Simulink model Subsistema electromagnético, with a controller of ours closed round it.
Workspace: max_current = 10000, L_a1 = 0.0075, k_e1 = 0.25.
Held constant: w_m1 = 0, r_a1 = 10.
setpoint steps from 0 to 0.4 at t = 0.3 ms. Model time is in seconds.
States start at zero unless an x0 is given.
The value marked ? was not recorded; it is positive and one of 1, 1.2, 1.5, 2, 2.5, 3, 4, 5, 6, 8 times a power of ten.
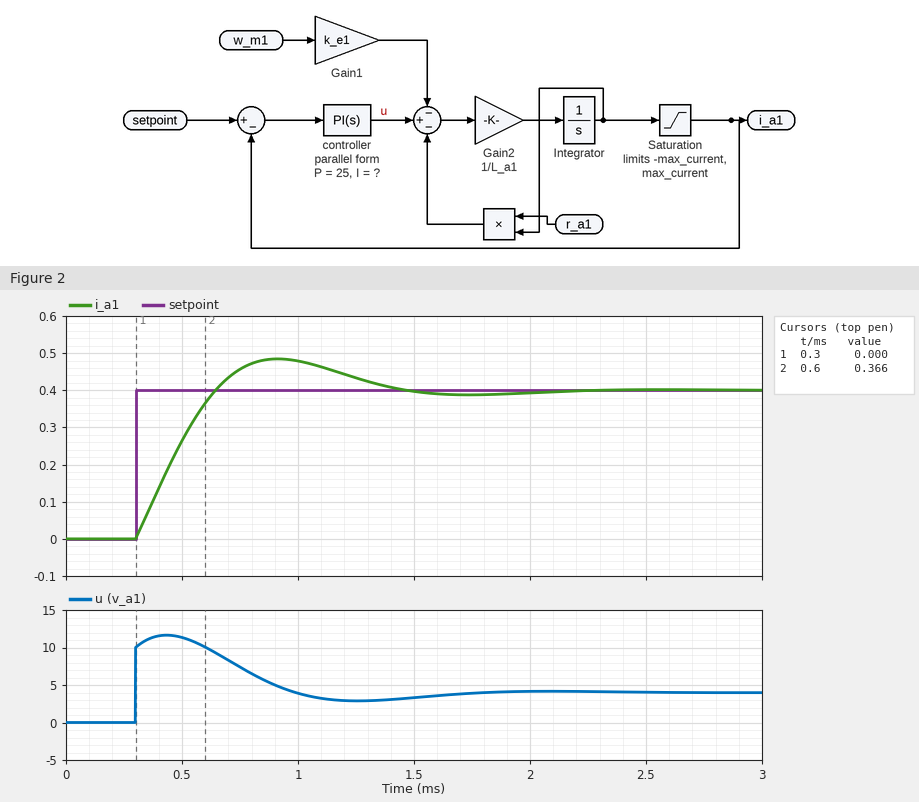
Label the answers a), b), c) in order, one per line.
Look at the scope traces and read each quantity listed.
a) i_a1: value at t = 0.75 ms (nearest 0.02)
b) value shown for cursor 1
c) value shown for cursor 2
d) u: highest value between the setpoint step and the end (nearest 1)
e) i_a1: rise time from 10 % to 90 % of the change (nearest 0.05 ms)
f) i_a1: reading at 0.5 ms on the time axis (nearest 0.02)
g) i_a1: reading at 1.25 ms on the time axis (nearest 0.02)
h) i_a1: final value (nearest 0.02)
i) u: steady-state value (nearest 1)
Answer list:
a) 0.46
b) 0.000
c) 0.366
d) 12
e) 0.25 ms
f) 0.26
g) 0.44
h) 0.40
i) 4
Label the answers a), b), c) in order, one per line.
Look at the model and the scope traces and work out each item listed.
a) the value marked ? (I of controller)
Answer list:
a) 150000
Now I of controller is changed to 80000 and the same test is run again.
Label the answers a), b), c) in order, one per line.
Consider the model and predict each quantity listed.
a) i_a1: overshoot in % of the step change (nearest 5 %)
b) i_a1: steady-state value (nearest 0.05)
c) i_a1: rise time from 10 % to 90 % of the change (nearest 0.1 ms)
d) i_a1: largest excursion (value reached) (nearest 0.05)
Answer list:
a) 10 %
b) 0.40
c) 0.4 ms
d) 0.45
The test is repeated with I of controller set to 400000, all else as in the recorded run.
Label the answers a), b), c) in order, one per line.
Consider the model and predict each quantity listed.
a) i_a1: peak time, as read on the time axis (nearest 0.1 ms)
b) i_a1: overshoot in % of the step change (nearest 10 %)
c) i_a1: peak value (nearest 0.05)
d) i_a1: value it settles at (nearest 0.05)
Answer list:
a) 0.7 ms
b) 40 %
c) 0.55
d) 0.40
